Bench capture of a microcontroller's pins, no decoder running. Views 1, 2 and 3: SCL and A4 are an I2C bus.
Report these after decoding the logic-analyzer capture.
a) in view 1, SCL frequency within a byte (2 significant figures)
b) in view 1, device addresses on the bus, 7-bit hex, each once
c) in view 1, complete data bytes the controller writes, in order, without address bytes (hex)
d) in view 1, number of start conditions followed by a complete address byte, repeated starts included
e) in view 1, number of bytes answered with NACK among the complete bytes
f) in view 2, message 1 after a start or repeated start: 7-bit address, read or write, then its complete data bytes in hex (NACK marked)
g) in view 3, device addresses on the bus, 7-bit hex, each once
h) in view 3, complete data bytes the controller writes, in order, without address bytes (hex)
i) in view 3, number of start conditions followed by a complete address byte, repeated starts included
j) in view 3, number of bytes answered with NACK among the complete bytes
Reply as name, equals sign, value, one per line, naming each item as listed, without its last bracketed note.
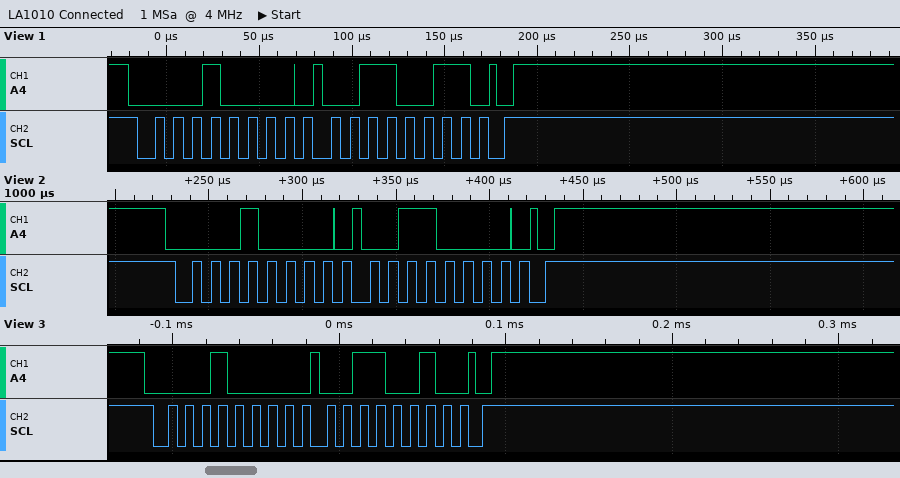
in view 1, SCL frequency within a byte = 100 kHz
in view 1, device addresses on the bus, 7-bit hex, each once = 0x08
in view 1, complete data bytes the controller writes, in order, without address bytes = 33
in view 1, number of start conditions followed by a complete address byte, repeated starts included = 1
in view 1, number of bytes answered with NACK among the complete bytes = 0
in view 2, message 1 after a start or repeated start: 7-bit address, read or write, then its complete data bytes in hex = 0x08 write: 30
in view 3, device addresses on the bus, 7-bit hex, each once = 0x08
in view 3, complete data bytes the controller writes, in order, without address bytes = 32
in view 3, number of start conditions followed by a complete address byte, repeated starts included = 1
in view 3, number of bytes answered with NACK among the complete bytes = 0
